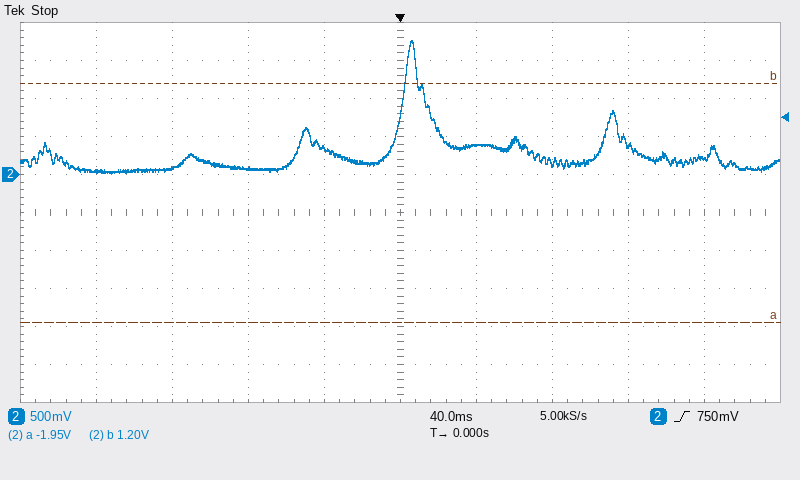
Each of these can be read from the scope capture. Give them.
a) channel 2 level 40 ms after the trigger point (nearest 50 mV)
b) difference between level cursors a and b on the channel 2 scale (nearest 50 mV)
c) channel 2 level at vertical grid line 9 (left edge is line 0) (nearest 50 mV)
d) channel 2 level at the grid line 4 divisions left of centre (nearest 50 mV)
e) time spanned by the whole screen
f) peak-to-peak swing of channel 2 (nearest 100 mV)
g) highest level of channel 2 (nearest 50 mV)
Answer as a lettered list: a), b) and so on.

a) 400 mV
b) 3.15 V
c) 200 mV
d) 50 mV
e) 400 ms
f) 1.70 V
g) 1.75 V
